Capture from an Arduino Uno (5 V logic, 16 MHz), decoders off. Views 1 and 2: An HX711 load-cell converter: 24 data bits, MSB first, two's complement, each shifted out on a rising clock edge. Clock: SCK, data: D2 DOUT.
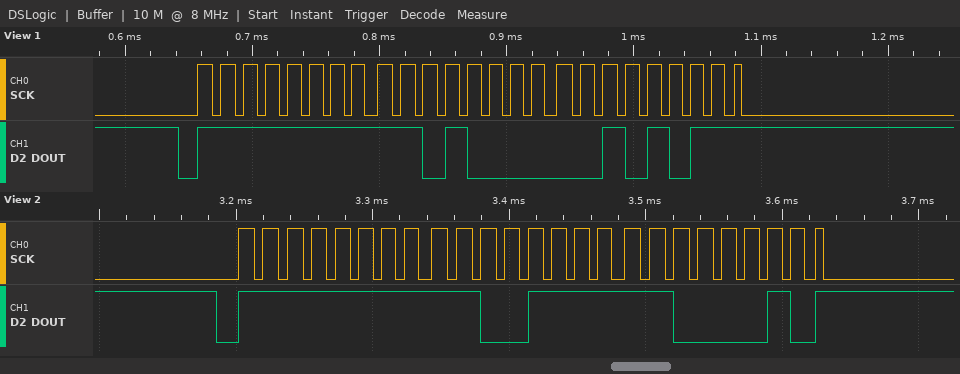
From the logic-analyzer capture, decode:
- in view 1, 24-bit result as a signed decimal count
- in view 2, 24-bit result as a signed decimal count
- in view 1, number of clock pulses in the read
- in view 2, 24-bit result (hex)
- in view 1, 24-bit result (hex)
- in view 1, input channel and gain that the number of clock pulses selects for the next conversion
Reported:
-12245
-12350
25
0xFFCFC2
0xFFD02B
channel A, gain 128
